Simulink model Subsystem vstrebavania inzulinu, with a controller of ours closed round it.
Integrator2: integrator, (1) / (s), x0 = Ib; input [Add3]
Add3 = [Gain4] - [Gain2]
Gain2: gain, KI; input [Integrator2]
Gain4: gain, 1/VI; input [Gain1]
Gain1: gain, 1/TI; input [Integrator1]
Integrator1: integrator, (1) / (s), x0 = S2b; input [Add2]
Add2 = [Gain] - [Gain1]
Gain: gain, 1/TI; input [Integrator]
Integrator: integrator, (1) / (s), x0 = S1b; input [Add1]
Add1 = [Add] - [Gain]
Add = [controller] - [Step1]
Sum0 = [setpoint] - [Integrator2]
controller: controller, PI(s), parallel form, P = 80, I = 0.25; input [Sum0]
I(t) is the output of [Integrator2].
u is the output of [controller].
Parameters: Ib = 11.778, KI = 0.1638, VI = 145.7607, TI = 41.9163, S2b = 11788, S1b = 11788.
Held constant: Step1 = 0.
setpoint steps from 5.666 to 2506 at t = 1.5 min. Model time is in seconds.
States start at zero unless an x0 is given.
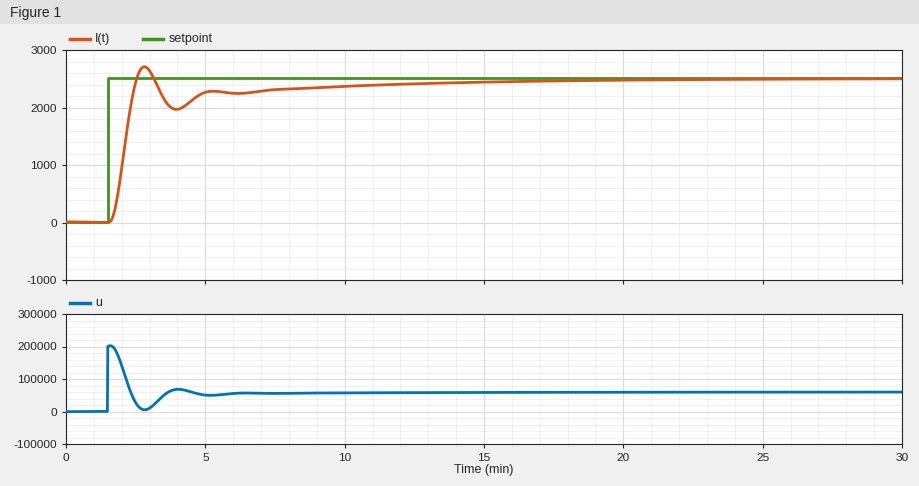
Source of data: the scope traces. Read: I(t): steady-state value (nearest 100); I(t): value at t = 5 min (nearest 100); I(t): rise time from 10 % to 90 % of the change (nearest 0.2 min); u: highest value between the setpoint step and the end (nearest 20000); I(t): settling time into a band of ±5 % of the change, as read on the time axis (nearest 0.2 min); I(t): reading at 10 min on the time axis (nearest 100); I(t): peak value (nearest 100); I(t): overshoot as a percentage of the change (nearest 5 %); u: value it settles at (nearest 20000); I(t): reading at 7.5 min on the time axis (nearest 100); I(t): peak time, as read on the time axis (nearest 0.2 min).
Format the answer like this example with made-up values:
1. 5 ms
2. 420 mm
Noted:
1. 2500
2. 2300
3. 0.6 min
4. 200000
5. 10.6 min
6. 2400
7. 2700
8. 10 %
9. 60000
10. 2300
11. 2.8 min
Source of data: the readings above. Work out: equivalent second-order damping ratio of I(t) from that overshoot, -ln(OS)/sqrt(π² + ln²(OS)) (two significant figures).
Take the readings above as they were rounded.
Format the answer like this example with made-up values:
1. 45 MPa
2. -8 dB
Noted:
1. 0.59
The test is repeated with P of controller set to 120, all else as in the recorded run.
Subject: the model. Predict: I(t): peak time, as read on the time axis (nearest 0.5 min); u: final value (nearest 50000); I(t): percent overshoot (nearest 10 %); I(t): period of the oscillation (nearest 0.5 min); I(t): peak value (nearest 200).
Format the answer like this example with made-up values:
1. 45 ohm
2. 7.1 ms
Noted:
1. 2.5 min
2. 50000
3. 20 %
4. 2.0 min
5. 3000
